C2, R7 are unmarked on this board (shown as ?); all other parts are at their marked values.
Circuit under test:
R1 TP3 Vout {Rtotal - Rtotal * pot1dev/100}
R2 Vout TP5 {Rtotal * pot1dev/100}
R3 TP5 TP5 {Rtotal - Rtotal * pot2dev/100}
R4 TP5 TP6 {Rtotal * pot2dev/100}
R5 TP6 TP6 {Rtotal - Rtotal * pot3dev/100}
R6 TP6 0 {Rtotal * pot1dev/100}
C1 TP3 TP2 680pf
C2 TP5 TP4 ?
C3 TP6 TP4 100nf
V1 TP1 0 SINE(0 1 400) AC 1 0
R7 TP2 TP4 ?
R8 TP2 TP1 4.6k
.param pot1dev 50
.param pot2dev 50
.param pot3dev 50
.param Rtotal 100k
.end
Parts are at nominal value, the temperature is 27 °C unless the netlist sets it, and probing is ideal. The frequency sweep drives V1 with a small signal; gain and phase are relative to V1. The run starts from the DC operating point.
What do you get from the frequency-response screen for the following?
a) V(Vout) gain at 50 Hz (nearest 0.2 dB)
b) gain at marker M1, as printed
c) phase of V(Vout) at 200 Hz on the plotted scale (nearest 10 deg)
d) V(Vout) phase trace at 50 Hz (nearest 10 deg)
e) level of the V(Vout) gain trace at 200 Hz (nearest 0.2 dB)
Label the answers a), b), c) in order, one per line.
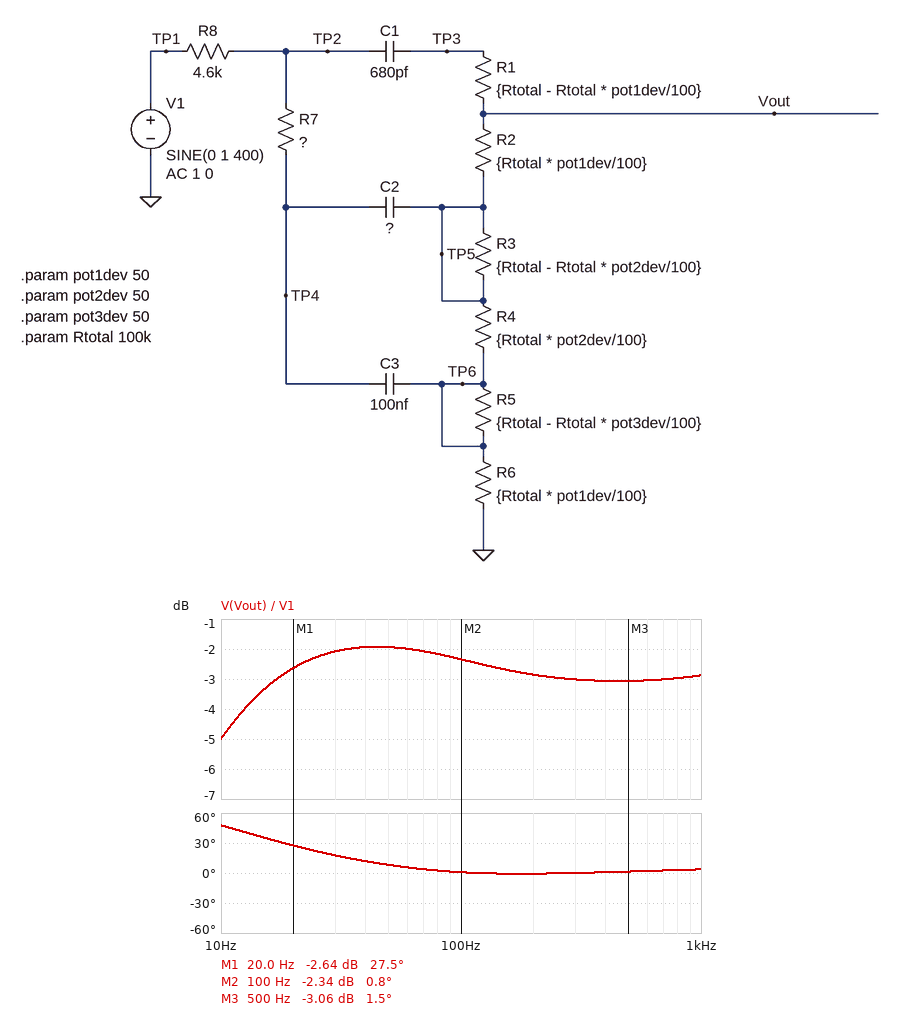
a) -2.0 dB
b) -2.64 dB
c) 0 deg
d) 10 deg
e) -2.8 dB
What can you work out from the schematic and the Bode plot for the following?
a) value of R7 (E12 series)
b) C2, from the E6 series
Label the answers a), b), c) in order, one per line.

a) 18 kΩ
b) 68 nF
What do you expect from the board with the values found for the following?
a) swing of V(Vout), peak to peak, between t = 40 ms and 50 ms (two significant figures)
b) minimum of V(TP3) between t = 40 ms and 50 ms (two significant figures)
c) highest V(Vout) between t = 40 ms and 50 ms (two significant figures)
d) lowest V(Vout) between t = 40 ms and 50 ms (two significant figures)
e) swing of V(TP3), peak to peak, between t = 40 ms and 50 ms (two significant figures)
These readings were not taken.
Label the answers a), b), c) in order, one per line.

a) 1.4 V
b) -710 mV
c) 700 mV
d) -700 mV
e) 1.4 V
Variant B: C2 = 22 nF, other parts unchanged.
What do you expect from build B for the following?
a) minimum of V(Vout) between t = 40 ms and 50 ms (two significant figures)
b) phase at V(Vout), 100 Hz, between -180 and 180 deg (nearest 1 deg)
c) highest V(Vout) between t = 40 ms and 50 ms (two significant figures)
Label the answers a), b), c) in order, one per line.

a) -720 mV
b) 7 deg
c) 720 mV
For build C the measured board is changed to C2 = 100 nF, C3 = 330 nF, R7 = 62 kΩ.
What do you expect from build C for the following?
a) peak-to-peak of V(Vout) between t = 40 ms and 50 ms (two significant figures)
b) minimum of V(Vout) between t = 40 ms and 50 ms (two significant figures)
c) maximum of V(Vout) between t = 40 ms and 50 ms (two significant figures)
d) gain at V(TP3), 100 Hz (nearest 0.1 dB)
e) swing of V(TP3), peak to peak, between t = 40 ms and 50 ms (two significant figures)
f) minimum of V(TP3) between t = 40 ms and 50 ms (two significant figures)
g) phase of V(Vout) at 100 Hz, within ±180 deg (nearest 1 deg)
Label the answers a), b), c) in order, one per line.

a) 900 mV
b) -450 mV
c) 450 mV
d) -7.0 dB
e) 940 mV
f) -470 mV
g) 0 deg
